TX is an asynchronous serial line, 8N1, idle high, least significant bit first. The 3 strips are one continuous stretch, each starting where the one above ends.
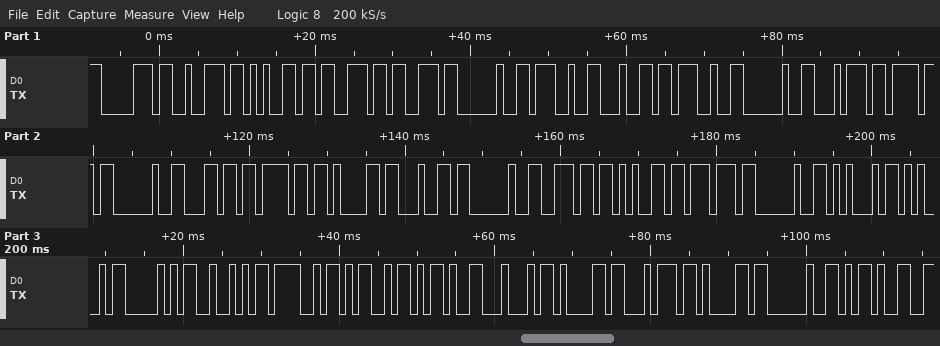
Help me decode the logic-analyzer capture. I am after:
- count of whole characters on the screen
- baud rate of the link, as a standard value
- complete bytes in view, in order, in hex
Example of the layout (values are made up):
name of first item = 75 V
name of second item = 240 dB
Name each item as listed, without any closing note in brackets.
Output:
count of whole characters on the screen = 35
baud rate of the link, as a standard value = 1200 baud
complete bytes in view, in order, in hex = 70 72 65 73 73 20 27 64 27 20 74 6F 20 6C 6F 61 64 20 6E 65 77 20 45 45 50 52 4F 4D 2D 44 61 74 61 20 2D
